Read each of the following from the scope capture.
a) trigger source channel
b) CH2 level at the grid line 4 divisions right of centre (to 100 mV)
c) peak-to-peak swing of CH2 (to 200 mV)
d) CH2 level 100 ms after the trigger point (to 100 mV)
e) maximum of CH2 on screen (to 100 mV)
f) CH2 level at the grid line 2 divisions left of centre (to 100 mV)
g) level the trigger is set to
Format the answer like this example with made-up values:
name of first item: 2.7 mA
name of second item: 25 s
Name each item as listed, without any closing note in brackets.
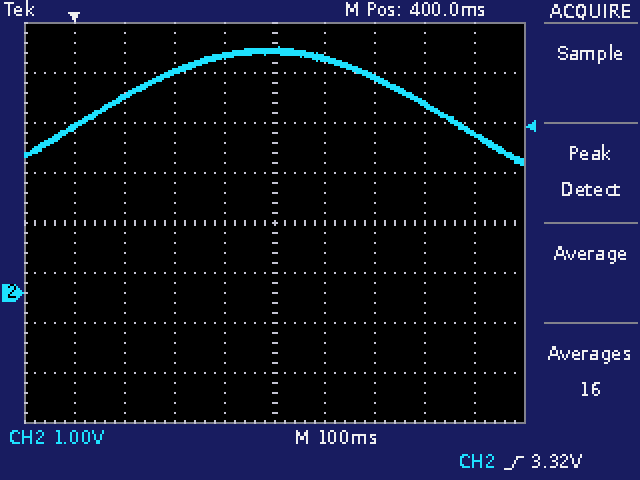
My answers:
trigger source channel: CH2
CH2 level at the grid line 4 divisions right of centre: 3.2 V
peak-to-peak swing of CH2: 2.4 V
CH2 level 100 ms after the trigger point: 3.9 V
maximum of CH2 on screen: 4.9 V
CH2 level at the grid line 2 divisions left of centre: 4.4 V
level the trigger is set to: 3.32 V
